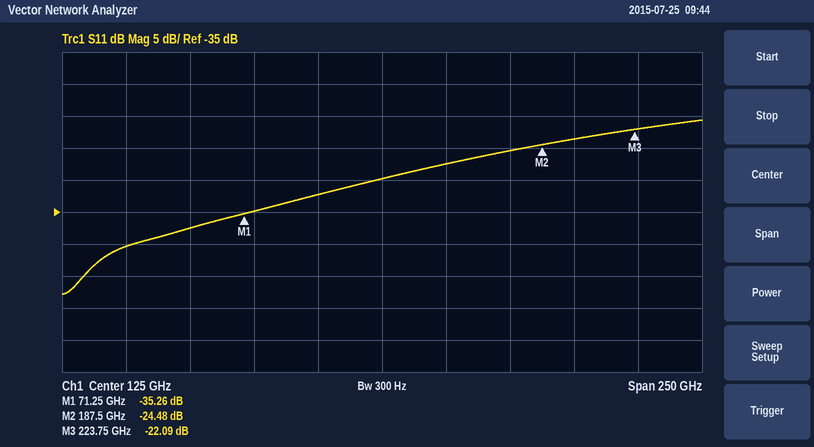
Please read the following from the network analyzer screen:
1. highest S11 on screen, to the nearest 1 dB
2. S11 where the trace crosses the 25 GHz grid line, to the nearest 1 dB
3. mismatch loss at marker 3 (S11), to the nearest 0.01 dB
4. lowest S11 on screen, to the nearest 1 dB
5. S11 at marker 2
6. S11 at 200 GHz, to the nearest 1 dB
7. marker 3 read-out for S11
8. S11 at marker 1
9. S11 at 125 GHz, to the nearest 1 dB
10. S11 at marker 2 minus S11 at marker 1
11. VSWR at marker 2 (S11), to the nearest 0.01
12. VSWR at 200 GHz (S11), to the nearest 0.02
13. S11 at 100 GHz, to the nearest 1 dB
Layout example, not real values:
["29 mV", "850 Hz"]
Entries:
["-21 dB", "-40 dB", "0.03 dB", "-48 dB", "-24.48 dB", "-24 dB", "-22.09 dB", "-35.26 dB", "-30 dB", "10.78 dB", "1.13", "1.14", "-32 dB"]
